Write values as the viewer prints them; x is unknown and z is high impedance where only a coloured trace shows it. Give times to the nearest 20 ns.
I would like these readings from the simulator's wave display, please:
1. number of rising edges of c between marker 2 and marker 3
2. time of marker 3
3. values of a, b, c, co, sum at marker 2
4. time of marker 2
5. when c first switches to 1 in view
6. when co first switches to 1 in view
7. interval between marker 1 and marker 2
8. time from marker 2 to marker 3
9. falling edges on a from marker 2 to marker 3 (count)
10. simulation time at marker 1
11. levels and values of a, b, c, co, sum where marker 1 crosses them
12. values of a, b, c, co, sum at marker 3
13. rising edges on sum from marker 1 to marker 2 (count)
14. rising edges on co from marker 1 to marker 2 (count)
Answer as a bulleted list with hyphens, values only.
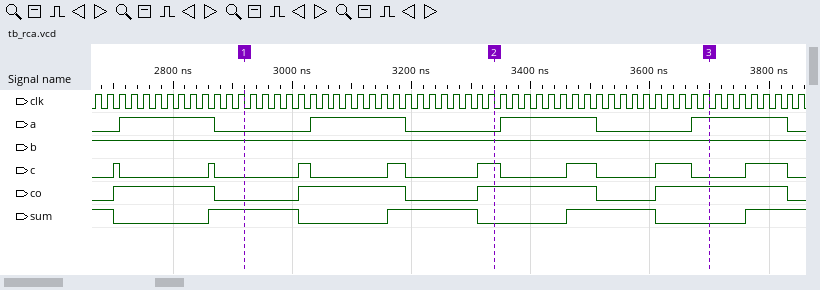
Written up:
- 2
- 3700 ns
- a=0, b=1, c=1, co=1, sum=0
- 3340 ns
- 2700 ns
- 2700 ns
- 420 ns
- 360 ns
- 1
- 2920 ns
- a=0, b=1, c=0, co=0, sum=1
- a=1, b=1, c=0, co=1, sum=0
- 1
- 2
